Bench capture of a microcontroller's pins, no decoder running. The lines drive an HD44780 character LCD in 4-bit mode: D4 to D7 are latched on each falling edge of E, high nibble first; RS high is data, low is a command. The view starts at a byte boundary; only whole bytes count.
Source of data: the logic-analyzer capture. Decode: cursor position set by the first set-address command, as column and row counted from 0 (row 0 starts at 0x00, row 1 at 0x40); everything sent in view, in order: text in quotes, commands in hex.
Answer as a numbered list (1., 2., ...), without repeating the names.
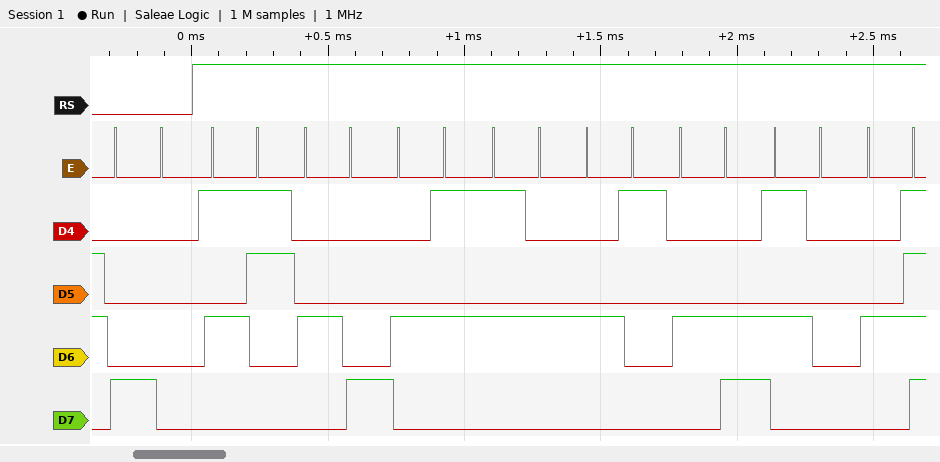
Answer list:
1. column 0, row 0
2. 0x80 "SHETALPO"
